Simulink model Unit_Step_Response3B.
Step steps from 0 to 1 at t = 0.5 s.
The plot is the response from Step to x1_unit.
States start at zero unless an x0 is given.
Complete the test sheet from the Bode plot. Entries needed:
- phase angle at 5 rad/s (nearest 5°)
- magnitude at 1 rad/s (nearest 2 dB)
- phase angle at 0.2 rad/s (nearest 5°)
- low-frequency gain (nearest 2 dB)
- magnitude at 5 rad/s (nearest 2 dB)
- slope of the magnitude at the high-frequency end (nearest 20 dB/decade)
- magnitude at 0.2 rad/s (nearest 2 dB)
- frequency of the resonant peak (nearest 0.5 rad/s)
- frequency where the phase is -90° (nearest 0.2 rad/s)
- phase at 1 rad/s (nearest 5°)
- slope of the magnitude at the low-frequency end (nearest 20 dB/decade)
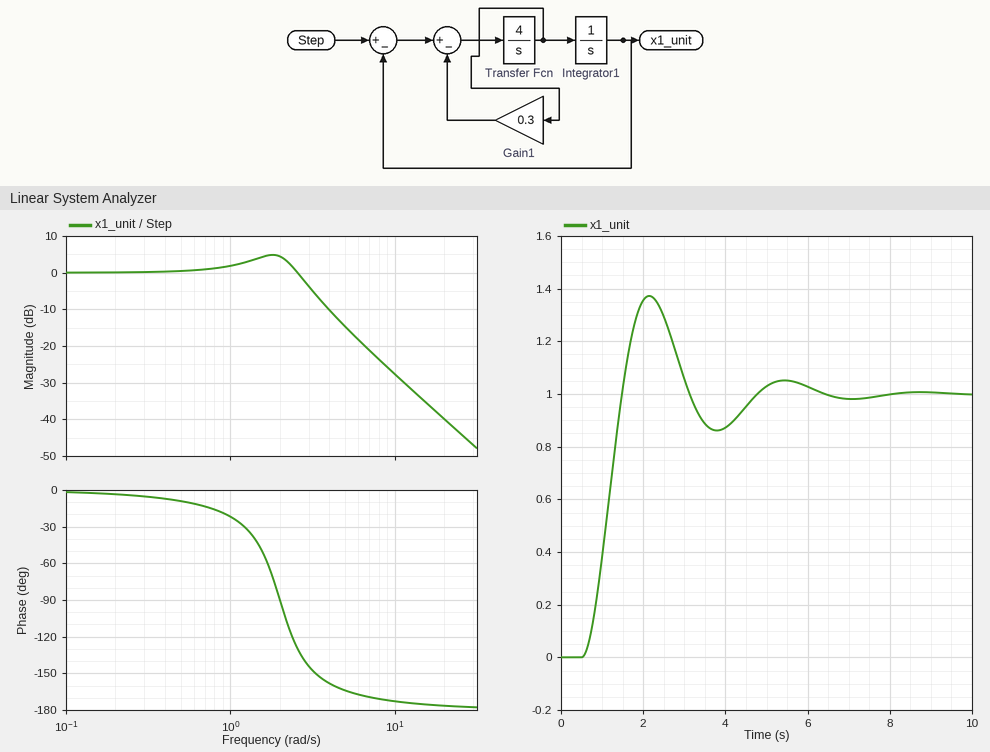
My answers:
-165°
2 dB
-5°
0 dB
-14 dB
-40 dB/decade
0 dB
2.0 rad/s
2.0 rad/s
-20°
0 dB/decade
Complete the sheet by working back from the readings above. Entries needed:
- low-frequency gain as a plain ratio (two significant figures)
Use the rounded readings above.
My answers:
1.0
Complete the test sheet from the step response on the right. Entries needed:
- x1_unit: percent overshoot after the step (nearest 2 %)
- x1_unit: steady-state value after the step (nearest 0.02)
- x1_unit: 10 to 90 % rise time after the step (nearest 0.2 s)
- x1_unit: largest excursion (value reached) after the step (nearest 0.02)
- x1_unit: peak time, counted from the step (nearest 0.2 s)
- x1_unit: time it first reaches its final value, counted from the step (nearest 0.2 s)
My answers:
38 %
1.00
0.6 s
1.38
1.6 s
1.0 s
